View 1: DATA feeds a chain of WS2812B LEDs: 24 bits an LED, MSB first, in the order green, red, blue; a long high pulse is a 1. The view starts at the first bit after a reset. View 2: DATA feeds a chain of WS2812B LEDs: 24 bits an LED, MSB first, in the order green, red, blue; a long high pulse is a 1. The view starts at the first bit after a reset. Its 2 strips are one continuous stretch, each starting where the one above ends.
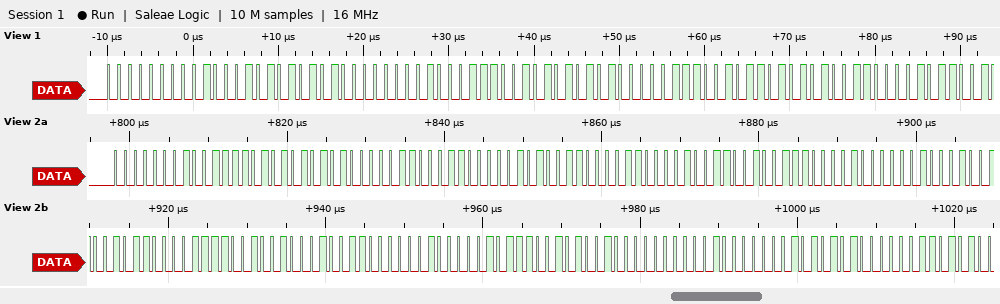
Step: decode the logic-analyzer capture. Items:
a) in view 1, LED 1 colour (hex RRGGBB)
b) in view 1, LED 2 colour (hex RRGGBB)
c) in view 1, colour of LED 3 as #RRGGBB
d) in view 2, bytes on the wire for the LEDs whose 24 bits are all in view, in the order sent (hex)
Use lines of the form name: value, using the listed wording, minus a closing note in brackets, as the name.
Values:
in view 1, LED 1 colour: #450054
in view 1, LED 2 colour: #390255
in view 1, colour of LED 3 as #RRGGBB: #2D0753
in view 2, bytes on the wire for the LEDs whose 24 bits are all in view, in the order sent: 01 3D 55 06 30 53 0C 26 4E 10 22 4B 0F 24 4C 08 2E 52 00 40 55
